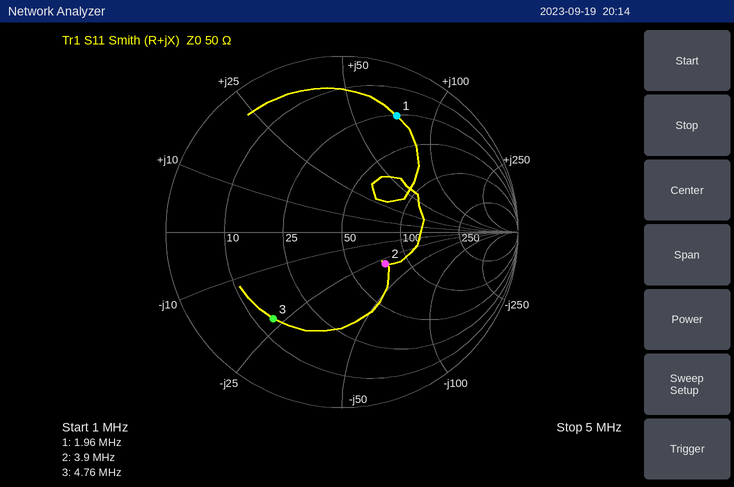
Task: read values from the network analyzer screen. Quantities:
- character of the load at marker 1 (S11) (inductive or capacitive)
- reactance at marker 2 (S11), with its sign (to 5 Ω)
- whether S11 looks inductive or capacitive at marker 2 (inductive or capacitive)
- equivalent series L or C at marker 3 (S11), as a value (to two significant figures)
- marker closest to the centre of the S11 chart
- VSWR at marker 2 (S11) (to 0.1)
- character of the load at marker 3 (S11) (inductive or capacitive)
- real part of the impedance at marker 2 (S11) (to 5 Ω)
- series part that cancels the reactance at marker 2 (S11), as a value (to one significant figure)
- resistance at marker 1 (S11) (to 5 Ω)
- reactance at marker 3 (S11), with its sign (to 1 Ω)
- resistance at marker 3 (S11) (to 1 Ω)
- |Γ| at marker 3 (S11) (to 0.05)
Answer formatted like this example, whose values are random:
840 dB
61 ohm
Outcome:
inductive
-30 Ω
capacitive
1.5 nF
marker 2
1.9
capacitive
75 Ω
1 µH
25 Ω
-23 Ω
14 Ω
0.65
